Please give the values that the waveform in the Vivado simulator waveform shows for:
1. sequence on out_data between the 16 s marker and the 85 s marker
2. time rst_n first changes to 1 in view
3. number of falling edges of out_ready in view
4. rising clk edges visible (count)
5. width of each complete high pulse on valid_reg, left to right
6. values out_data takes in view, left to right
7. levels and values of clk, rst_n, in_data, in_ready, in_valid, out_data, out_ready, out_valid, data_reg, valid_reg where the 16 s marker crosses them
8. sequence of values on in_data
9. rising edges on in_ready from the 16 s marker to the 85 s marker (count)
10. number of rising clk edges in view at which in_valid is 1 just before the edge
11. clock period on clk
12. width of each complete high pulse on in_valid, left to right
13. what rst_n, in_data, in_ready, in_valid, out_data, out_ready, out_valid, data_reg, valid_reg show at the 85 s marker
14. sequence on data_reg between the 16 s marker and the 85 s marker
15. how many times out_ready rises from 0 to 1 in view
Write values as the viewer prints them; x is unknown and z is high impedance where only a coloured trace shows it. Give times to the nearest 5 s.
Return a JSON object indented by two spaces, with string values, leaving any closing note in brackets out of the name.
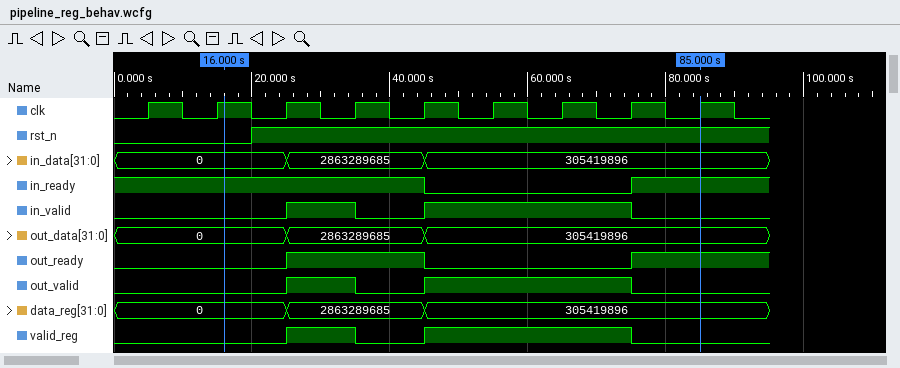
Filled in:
{
  "sequence on out_data between the 16 s marker and the 85 s marker": "0, 2863289685, 305419896",
  "time rst_n first changes to 1 in view": "20 s",
  "number of falling edges of out_ready in view": "1",
  "rising clk edges visible": "9",
  "width of each complete high pulse on valid_reg, left to right": "10 s, 30 s",
  "values out_data takes in view, left to right": "0, 2863289685, 305419896",
  "levels and values of clk, rst_n, in_data, in_ready, in_valid, out_data, out_ready, out_valid, data_reg, valid_reg where the 16 s marker crosses them": "clk=1, rst_n=0, in_data=0, in_ready=1, in_valid=0, out_data=0, out_ready=0, out_valid=0, data_reg=0, valid_reg=0",
  "sequence of values on in_data": "0, 2863289685, 305419896",
  "rising edges on in_ready from the 16 s marker to the 85 s marker": "1",
  "number of rising clk edges in view at which in_valid is 1 just before the edge": "4",
  "clock period on clk": "10 s",
  "width of each complete high pulse on in_valid, left to right": "10 s, 30 s",
  "what rst_n, in_data, in_ready, in_valid, out_data, out_ready, out_valid, data_reg, valid_reg show at the 85 s marker": "rst_n=1, in_data=305419896, in_ready=1, in_valid=0, out_data=305419896, out_ready=1, out_valid=0, data_reg=305419896, valid_reg=0",
  "sequence on data_reg between the 16 s marker and the 85 s marker": "0, 2863289685, 305419896",
  "how many times out_ready rises from 0 to 1 in view": "2"
}
